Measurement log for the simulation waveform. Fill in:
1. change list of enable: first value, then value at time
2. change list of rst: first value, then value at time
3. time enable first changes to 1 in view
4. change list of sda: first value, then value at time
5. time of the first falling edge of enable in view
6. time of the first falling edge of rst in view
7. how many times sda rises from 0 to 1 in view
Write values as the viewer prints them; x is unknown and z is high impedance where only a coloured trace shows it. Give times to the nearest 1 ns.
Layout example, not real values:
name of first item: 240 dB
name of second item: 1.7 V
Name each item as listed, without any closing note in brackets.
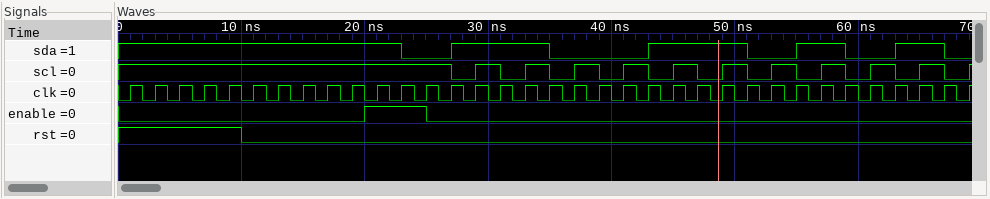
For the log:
change list of enable: first value, then value at time: 0, 1 at 20 ns, 0 at 25 ns
change list of rst: first value, then value at time: 1, 0 at 10 ns
time enable first changes to 1 in view: 20 ns
change list of sda: first value, then value at time: 1, 0 at 23 ns, 1 at 27 ns, 0 at 35 ns, 1 at 43 ns, 0 at 51 ns, 1 at 55 ns, 0 at 59 ns, 1 at 63 ns, 0 at 67 ns
time of the first falling edge of enable in view: 25 ns
time of the first falling edge of rst in view: 10 ns
how many times sda rises from 0 to 1 in view: 4
